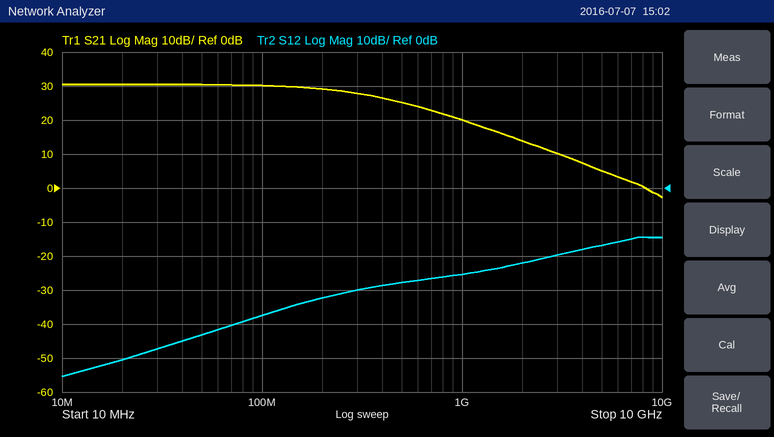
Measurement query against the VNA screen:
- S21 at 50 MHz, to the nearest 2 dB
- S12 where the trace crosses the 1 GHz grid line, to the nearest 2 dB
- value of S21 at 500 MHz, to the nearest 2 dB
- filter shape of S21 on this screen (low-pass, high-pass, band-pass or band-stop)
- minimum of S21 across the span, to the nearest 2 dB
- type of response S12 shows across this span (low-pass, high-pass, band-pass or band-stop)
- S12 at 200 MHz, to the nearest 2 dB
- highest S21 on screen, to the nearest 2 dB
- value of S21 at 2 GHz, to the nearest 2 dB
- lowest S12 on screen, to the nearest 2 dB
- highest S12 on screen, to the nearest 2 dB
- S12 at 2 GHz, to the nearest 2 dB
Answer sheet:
30 dB
-26 dB
26 dB
low-pass
-2 dB
high-pass
-32 dB
30 dB
14 dB
-56 dB
-14 dB
-22 dB
